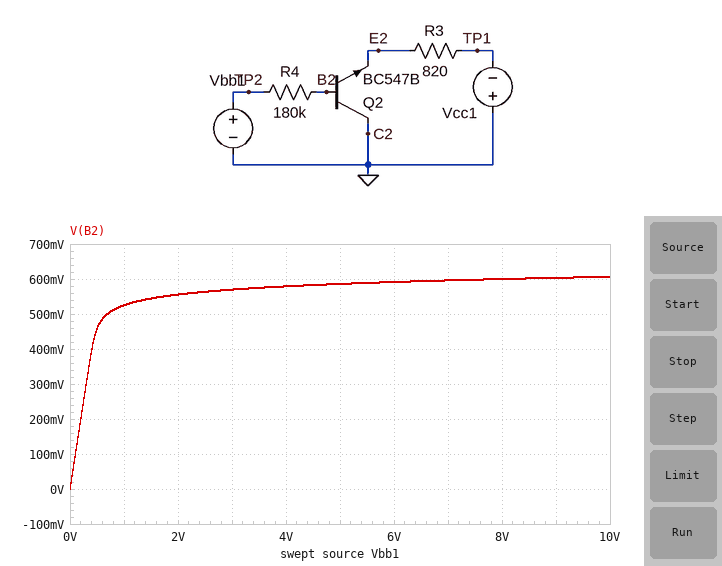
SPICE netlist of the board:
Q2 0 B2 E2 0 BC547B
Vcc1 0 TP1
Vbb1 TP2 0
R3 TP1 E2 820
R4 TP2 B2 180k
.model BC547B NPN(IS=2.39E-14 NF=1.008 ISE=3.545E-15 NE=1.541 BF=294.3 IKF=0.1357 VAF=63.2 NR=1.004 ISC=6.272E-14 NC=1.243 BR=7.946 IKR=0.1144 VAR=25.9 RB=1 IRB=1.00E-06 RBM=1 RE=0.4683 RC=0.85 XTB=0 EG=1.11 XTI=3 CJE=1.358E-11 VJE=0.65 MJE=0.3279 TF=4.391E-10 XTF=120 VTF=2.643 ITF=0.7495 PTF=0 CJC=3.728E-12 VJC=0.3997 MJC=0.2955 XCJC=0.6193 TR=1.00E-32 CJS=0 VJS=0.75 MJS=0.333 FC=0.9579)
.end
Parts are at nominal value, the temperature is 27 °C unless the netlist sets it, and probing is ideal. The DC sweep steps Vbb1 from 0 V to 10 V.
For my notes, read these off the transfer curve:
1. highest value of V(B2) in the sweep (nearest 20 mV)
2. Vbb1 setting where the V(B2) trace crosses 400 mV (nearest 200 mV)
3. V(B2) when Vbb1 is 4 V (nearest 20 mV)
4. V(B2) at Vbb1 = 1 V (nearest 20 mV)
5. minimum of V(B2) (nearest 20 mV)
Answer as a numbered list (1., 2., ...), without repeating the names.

1. 600 mV
2. 400 mV
3. 580 mV
4. 520 mV
5. 0 V
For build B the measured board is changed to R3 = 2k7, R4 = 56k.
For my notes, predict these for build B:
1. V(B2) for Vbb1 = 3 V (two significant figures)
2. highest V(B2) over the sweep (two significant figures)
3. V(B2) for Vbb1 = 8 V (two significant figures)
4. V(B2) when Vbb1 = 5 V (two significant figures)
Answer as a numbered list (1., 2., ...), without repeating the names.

1. 600 mV
2. 640 mV
3. 630 mV
4. 620 mV
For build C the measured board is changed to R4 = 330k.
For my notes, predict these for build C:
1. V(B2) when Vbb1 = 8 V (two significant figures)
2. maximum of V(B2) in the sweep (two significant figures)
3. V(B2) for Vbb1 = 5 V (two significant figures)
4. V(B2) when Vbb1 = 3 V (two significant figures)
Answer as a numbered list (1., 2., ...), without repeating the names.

1. 580 mV
2. 590 mV
3. 570 mV
4. 550 mV
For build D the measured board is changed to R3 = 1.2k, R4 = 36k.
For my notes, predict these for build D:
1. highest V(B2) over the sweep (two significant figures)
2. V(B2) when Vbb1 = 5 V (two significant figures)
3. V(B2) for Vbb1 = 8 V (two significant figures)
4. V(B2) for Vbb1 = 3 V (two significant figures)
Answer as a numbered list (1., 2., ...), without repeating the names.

1. 650 mV
2. 630 mV
3. 640 mV
4. 610 mV
